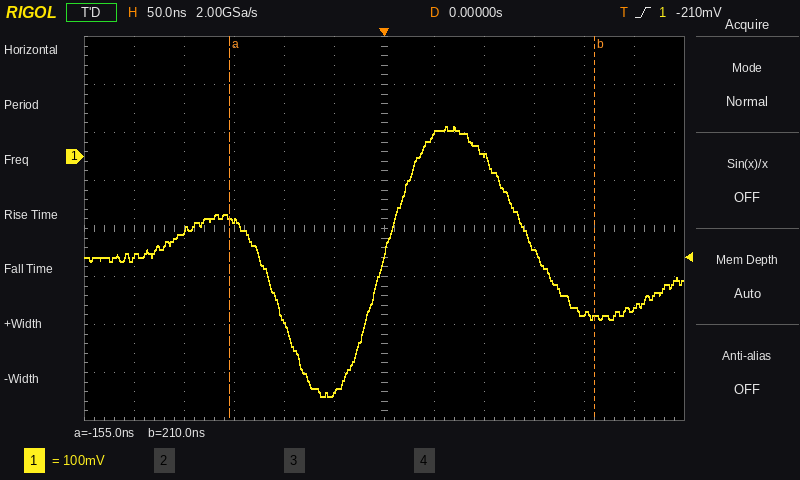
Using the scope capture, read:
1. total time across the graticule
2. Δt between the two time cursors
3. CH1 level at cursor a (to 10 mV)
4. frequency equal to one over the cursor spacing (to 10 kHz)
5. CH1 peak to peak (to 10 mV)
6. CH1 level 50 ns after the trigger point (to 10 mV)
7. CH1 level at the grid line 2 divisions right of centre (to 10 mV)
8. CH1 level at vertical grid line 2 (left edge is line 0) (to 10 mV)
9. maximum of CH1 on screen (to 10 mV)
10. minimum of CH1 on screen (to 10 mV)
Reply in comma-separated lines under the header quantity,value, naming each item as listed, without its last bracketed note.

quantity,value
total time across the graticule,600 ns
Δt between the two time cursors,365 ns
CH1 level at cursor a,-130 mV
frequency equal to one over the cursor spacing,2.74 MHz
CH1 peak to peak,560 mV
CH1 level 50 ns after the trigger point,50 mV
CH1 level at the grid line 2 divisions right of centre,0 mV
CH1 level at vertical grid line 2 (left edge is line 0),-150 mV
maximum of CH1 on screen,60 mV
minimum of CH1 on screen,-500 mV
